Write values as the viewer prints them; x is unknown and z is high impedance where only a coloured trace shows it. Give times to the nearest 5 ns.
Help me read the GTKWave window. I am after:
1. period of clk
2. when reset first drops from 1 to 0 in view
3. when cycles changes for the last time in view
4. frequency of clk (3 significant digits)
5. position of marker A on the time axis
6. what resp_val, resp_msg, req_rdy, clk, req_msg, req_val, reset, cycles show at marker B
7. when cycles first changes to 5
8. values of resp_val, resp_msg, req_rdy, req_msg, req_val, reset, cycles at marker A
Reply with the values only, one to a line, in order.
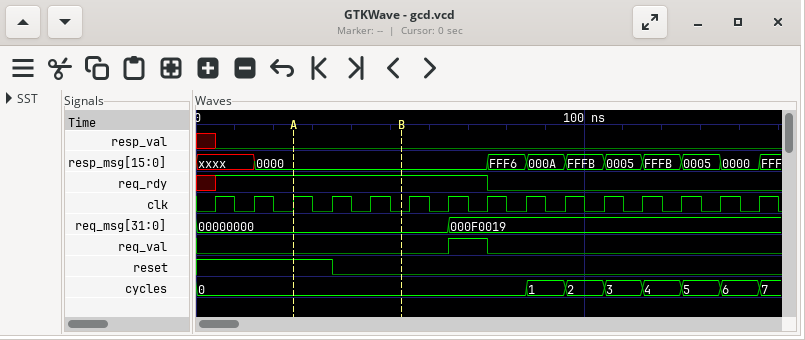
10 ns
35 ns
145 ns
100 MHz
25 ns
resp_val=0, resp_msg=0000, req_rdy=1, clk=0, req_msg=00000000, req_val=0, reset=0, cycles=0
125 ns
resp_val=0, resp_msg=0000, req_rdy=1, req_msg=00000000, req_val=0, reset=1, cycles=0
